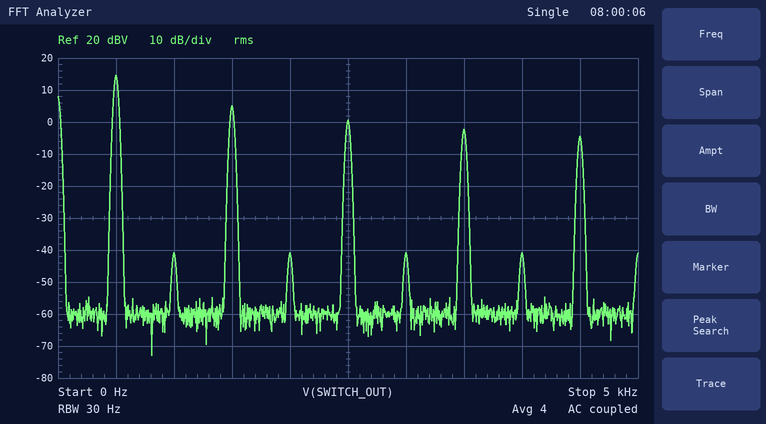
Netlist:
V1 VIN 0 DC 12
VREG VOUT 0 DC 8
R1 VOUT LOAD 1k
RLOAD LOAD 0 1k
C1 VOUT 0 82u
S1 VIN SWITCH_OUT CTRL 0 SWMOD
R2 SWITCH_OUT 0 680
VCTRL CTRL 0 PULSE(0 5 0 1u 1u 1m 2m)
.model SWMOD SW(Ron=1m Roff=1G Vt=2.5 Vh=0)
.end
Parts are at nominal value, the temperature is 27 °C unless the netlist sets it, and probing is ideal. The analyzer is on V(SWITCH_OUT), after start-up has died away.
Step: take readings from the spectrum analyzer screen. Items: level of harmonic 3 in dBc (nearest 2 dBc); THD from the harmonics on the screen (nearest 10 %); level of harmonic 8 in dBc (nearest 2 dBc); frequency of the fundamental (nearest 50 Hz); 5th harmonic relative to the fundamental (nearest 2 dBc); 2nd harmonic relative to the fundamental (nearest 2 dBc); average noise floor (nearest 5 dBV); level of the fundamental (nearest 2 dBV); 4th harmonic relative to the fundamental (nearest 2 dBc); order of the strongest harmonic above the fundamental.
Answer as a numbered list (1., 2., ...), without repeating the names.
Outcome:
1. -10 dBc
2. 40 %
3. -56 dBc
4. 500 Hz
5. -14 dBc
6. -56 dBc
7. -60 dBV
8. 14 dBV
9. -56 dBc
10. 3
